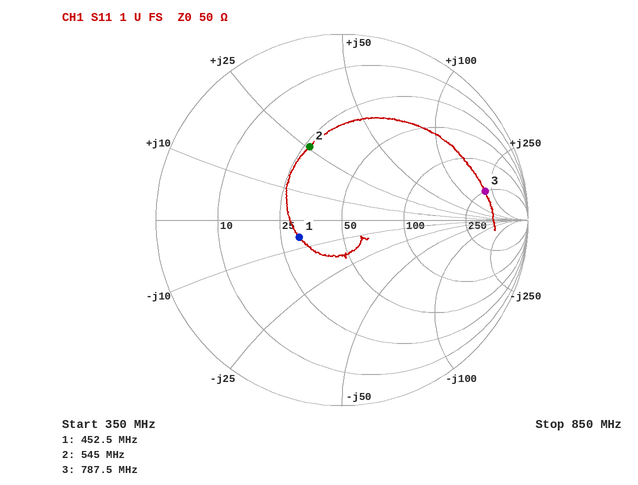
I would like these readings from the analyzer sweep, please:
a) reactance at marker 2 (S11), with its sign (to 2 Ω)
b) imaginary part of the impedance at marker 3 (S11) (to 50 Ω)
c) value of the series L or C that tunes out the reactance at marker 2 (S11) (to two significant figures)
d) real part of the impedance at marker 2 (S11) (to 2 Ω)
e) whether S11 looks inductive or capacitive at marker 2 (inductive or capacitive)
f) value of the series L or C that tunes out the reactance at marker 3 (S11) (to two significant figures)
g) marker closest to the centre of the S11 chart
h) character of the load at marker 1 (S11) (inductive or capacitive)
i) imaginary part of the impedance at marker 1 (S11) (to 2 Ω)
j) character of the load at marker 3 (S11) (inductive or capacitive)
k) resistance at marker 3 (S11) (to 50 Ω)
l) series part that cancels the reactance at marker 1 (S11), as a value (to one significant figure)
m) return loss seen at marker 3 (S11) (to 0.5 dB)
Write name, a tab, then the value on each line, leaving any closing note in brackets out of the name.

reactance at marker 2 (S11), with its sign	+26 Ω
imaginary part of the impedance at marker 3 (S11)	+200 Ω
value of the series L or C that tunes out the reactance at marker 2 (S11)	11 pF
real part of the impedance at marker 2 (S11)	26 Ω
whether S11 looks inductive or capacitive at marker 2	inductive
value of the series L or C that tunes out the reactance at marker 3 (S11)	1.0 pF
marker closest to the centre of the S11 chart	marker 1
character of the load at marker 1 (S11)	capacitive
imaginary part of the impedance at marker 1 (S11)	-6 Ω
character of the load at marker 3 (S11)	inductive
resistance at marker 3 (S11)	250 Ω
series part that cancels the reactance at marker 1 (S11), as a value	2 nH
return loss seen at marker 3 (S11)	2.0 dB
